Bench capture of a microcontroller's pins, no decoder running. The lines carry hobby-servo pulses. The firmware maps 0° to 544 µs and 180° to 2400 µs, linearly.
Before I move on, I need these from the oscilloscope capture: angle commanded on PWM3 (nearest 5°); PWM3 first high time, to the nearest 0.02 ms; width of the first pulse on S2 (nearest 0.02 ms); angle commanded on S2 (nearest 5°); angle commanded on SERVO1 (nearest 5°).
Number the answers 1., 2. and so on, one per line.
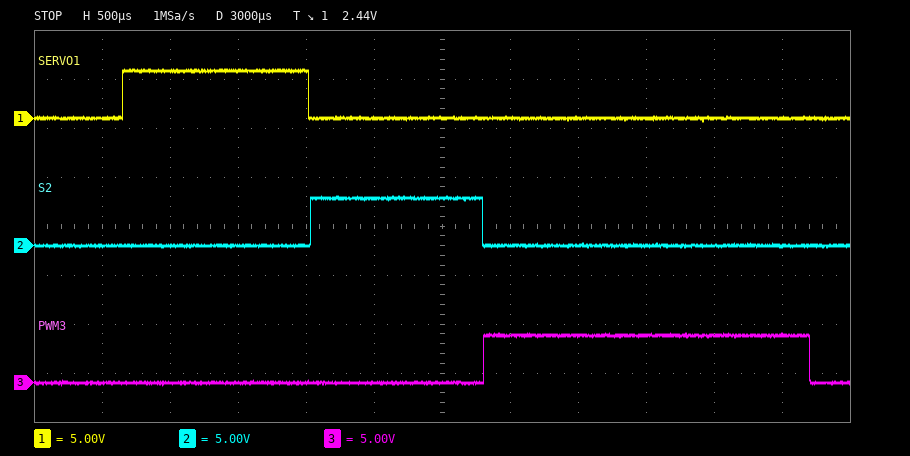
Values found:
1. 180°
2. 2.40 ms
3. 1.26 ms
4. 70°
5. 80°
